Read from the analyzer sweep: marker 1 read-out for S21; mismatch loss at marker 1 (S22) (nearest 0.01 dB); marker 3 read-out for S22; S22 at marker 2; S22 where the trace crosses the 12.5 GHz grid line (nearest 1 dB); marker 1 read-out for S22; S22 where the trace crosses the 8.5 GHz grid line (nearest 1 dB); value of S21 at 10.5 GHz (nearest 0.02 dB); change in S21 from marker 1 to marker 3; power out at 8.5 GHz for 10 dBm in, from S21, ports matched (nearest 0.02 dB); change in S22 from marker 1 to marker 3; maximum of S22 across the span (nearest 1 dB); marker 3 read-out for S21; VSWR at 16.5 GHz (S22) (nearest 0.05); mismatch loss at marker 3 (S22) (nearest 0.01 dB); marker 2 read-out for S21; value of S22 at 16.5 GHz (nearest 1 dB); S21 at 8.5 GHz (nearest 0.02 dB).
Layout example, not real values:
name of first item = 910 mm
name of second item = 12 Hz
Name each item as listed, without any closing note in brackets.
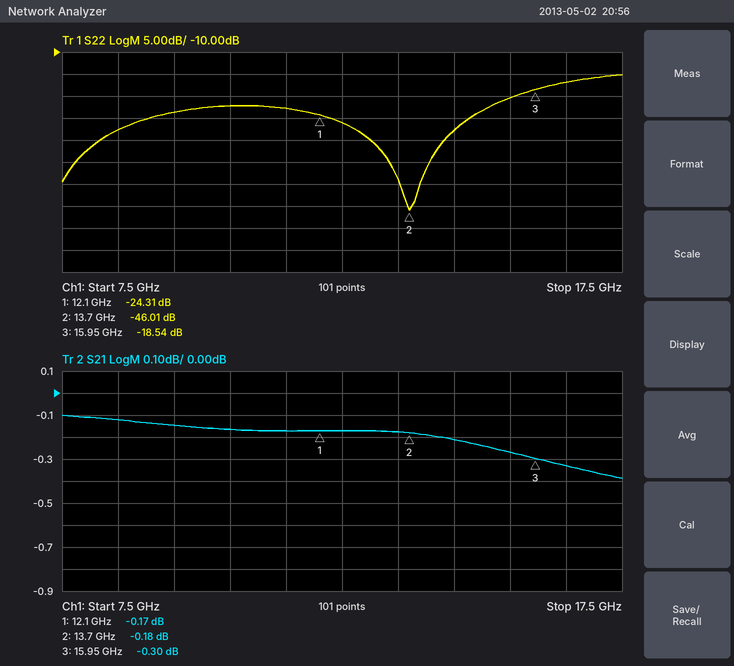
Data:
marker 1 read-out for S21 = -0.17 dB
mismatch loss at marker 1 (S22) = 0.02 dB
marker 3 read-out for S22 = -18.54 dB
S22 at marker 2 = -46.01 dB
S22 where the trace crosses the 12.5 GHz grid line = -26 dB
marker 1 read-out for S22 = -24.31 dB
S22 where the trace crosses the 8.5 GHz grid line = -28 dB
value of S21 at 10.5 GHz = -0.16 dB
change in S21 from marker 1 to marker 3 = -0.13 dB
power out at 8.5 GHz for 10 dBm in, from S21, ports matched = 9.88 dBm
change in S22 from marker 1 to marker 3 = 5.77 dB
maximum of S22 across the span = -15 dB
marker 3 read-out for S21 = -0.30 dB
VSWR at 16.5 GHz (S22) = 1.35
mismatch loss at marker 3 (S22) = 0.06 dB
marker 2 read-out for S21 = -0.18 dB
value of S22 at 16.5 GHz = -17 dB
S21 at 8.5 GHz = -0.12 dB
